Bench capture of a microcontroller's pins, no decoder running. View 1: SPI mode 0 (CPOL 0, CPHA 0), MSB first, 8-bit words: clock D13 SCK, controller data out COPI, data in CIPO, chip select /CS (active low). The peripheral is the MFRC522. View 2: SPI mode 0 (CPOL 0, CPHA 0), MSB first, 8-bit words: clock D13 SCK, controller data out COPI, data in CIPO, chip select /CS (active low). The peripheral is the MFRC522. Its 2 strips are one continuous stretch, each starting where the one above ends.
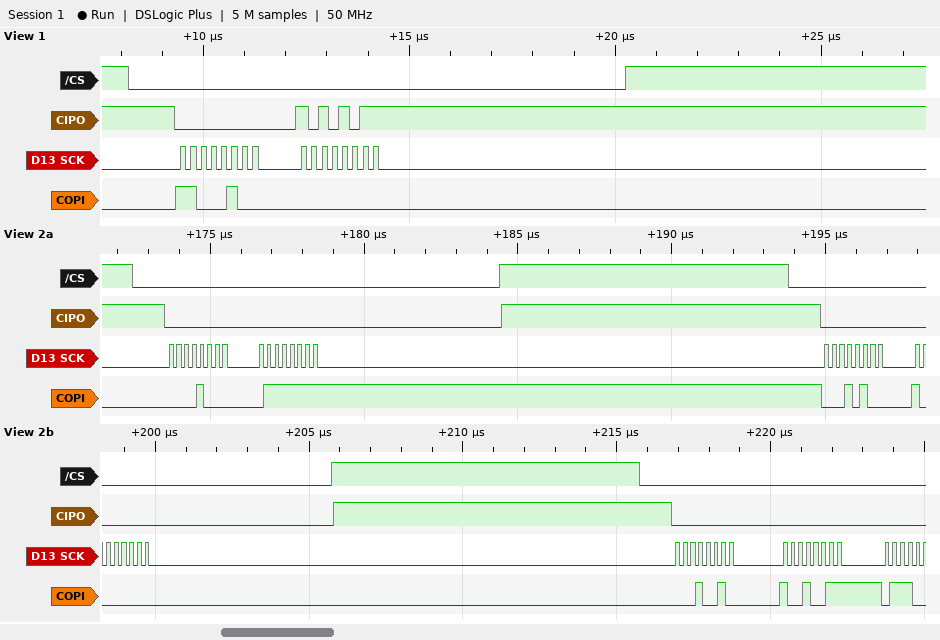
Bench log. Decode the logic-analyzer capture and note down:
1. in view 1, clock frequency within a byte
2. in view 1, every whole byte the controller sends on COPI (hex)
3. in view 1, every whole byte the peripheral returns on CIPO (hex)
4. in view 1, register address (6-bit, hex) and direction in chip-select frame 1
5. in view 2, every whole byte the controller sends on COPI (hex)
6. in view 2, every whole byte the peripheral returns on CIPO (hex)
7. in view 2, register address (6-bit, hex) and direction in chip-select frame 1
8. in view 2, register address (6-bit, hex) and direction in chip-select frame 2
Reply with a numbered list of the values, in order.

1. 4 MHz
2. C4 00
3. 00 AB
4. 0x22 read
5. 08 7F 14 80 12 93
6. 00 00 00 00 00 00
7. 0x04 write
8. 0x0A write
